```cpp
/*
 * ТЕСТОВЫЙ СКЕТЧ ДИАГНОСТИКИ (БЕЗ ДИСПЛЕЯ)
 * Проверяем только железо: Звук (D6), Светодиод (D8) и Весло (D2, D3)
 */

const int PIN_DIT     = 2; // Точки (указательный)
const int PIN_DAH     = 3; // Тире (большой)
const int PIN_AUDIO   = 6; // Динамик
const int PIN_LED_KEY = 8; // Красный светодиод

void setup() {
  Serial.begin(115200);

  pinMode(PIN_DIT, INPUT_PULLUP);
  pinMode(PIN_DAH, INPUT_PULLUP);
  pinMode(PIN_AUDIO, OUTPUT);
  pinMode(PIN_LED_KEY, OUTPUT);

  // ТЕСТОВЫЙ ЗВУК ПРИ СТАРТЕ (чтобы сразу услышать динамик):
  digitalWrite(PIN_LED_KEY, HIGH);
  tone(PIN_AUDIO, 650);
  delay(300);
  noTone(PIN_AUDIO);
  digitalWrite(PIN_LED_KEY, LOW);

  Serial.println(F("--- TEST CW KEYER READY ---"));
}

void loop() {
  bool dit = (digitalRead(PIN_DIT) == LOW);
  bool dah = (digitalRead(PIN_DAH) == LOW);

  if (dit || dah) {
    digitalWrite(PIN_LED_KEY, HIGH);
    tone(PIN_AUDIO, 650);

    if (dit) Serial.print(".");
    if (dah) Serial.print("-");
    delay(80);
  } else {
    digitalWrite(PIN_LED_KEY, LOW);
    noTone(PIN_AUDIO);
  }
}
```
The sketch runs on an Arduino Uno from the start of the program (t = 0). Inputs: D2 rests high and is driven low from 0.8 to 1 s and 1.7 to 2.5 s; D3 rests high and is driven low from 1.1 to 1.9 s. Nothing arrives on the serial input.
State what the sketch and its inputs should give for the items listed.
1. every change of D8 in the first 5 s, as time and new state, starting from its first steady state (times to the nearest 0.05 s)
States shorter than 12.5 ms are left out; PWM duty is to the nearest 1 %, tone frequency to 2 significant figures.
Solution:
0 s high; 0.3 s low; 0.8 s high; 1.05 s low; 1.1 s high; 2.55 s low
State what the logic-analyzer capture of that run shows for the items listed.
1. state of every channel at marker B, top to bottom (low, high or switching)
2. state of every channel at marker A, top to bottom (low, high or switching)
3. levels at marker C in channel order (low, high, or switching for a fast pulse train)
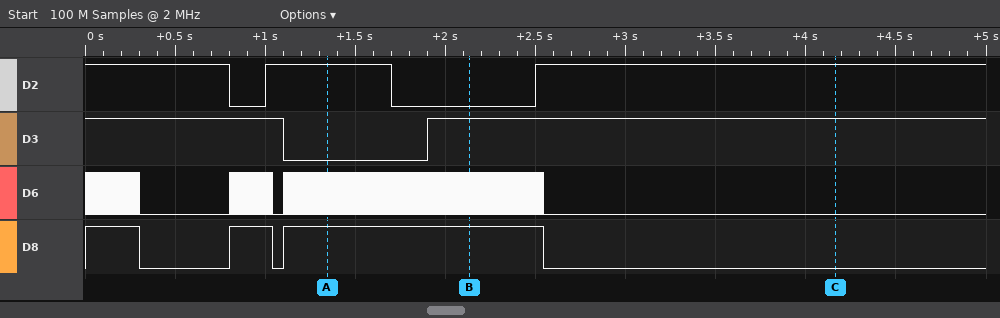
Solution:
D2 low, D3 high, D6 switching, D8 high
D2 high, D3 low, D6 switching, D8 high
D2 high, D3 high, D6 low, D8 low
